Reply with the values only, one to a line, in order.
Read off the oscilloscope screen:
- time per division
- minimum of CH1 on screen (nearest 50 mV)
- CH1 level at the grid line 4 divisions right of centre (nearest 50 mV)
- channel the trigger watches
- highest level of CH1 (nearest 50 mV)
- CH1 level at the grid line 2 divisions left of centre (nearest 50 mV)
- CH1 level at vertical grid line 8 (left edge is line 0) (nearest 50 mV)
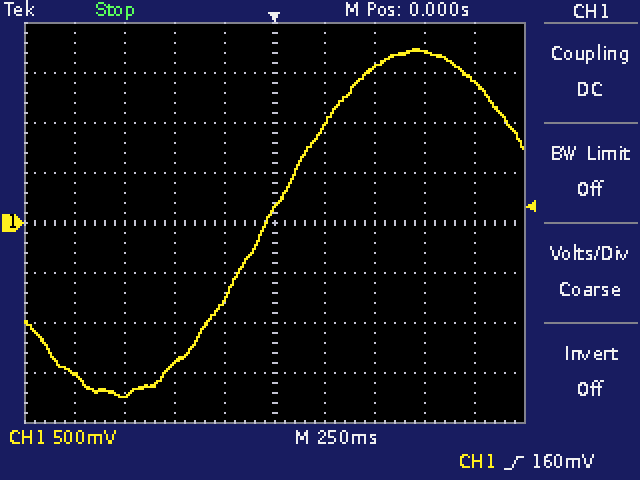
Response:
250 ms
-1.75 V
1.40 V
CH1
1.75 V
-1.40 V
1.70 V
